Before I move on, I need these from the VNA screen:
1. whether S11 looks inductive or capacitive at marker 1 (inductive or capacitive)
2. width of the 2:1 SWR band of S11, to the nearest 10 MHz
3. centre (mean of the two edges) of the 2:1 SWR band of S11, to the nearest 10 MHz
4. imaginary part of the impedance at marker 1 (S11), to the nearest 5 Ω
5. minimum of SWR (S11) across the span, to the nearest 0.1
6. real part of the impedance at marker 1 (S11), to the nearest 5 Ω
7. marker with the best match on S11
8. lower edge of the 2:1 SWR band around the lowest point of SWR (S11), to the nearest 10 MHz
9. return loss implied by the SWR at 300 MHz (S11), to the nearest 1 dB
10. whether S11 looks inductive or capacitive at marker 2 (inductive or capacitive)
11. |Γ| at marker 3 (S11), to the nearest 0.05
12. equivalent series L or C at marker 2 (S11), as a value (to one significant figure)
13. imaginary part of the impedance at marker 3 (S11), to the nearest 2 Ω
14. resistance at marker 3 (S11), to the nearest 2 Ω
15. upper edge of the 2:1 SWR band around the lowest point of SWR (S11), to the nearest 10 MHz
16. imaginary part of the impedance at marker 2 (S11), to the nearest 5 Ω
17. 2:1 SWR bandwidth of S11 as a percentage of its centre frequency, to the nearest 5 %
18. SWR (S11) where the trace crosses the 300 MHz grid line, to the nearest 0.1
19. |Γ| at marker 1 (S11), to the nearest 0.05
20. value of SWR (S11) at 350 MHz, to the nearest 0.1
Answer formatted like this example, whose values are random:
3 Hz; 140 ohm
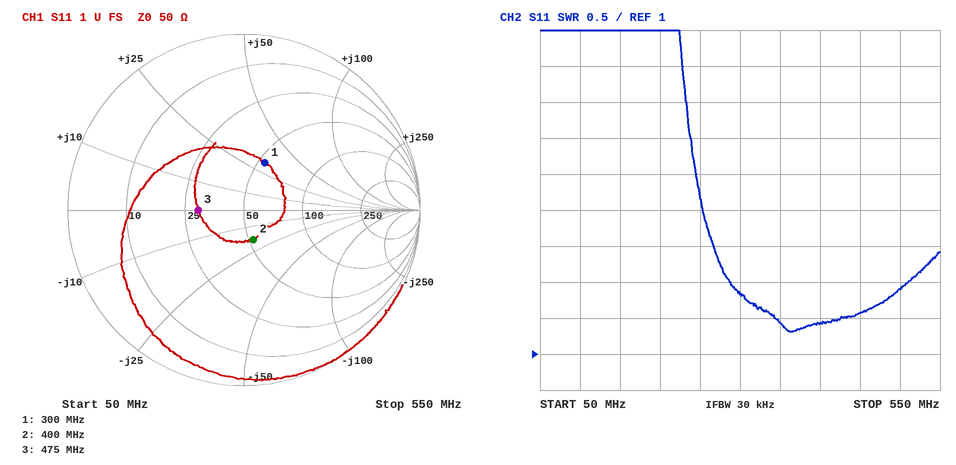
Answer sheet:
inductive; 220 MHz; 400 MHz; +30 Ω; 1.3; 55 Ω; marker 2; 290 MHz; 11 dB; capacitive; 0.25; 20 pF; 0 Ω; 30 Ω; 510 MHz; -20 Ω; 55 %; 1.8; 0.30; 1.4
